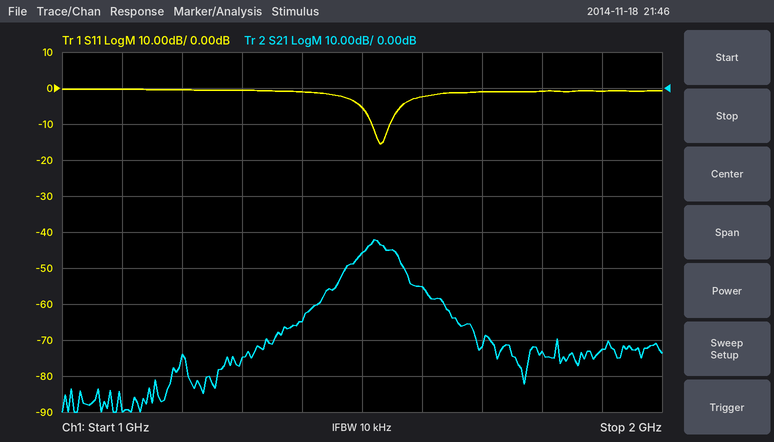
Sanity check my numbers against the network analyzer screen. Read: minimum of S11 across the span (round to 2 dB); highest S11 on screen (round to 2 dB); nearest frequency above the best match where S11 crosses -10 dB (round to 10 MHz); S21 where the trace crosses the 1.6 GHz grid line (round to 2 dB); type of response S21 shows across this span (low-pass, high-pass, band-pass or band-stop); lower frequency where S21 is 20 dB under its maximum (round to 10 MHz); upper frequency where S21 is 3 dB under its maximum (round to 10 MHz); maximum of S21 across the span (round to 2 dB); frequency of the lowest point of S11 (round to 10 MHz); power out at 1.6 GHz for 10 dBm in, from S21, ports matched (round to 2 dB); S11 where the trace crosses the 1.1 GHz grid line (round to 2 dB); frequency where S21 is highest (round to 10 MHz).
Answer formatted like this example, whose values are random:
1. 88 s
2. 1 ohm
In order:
1. -16 dB
2. 0 dB
3. 1.55 GHz
4. -56 dB
5. band-pass
6. 1.41 GHz
7. 1.55 GHz
8. -42 dB
9. 1.53 GHz
10. -46 dBm
11. 0 dB
12. 1.52 GHz
